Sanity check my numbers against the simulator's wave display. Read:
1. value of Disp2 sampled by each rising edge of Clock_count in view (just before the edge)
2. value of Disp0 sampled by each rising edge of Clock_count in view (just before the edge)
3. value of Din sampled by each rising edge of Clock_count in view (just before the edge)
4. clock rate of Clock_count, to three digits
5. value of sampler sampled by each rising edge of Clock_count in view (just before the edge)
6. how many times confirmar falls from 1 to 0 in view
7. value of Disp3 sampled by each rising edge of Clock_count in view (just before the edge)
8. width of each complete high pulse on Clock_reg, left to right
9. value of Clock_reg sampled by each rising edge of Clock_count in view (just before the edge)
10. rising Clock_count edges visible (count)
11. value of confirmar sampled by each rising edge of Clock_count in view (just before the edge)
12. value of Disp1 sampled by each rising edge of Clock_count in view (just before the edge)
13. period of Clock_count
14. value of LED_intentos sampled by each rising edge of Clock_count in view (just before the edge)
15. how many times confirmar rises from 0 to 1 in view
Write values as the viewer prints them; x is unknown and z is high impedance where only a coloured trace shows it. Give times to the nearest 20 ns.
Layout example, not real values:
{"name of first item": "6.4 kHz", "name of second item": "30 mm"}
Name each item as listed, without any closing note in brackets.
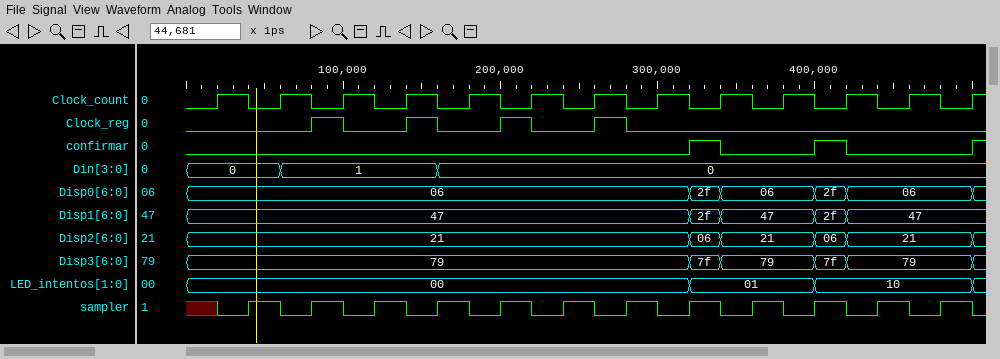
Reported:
{"value of Disp2 sampled by each rising edge of Clock_count in view": "21, 21, 21, 21, 21, 21, 21, 21, 06, 21, 06, 21, 21", "value of Disp0 sampled by each rising edge of Clock_count in view": "06, 06, 06, 06, 06, 06, 06, 06, 2f, 06, 2f, 06, 06", "value of Din sampled by each rising edge of Clock_count in view": "0, 0, 1, 1, 0, 0, 0, 0, 0, 0, 0, 0, 0", "clock rate of Clock_count, to three digits": "25.0 MHz", "value of sampler sampled by each rising edge of Clock_count in view": "x 1 1 1 1 1 1 1 1 1 1 1 1", "how many times confirmar falls from 1 to 0 in view": "2", "value of Disp3 sampled by each rising edge of Clock_count in view": "79, 79, 79, 79, 79, 79, 79, 79, 7f, 79, 7f, 79, 79", "width of each complete high pulse on Clock_reg, left to right": "20 ns, 20 ns, 20 ns, 20 ns", "value of Clock_reg sampled by each rising edge of Clock_count in view": "0 0 1 0 0 1 0 0 0 0 0 0 0", "rising Clock_count edges visible": "13", "value of confirmar sampled by each rising edge of Clock_count in view": "0 0 0 0 0 0 0 0 1 0 1 0 0", "value of Disp1 sampled by each rising edge of Clock_count in view": "47, 47, 47, 47, 47, 47, 47, 47, 2f, 47, 2f, 47, 47", "period of Clock_count": "40 ns", "value of LED_intentos sampled by each rising edge of Clock_count in view": "00, 00, 00, 00, 00, 00, 00, 00, 01, 01, 10, 10, 10", "how many times confirmar rises from 0 to 1 in view": "3"}
